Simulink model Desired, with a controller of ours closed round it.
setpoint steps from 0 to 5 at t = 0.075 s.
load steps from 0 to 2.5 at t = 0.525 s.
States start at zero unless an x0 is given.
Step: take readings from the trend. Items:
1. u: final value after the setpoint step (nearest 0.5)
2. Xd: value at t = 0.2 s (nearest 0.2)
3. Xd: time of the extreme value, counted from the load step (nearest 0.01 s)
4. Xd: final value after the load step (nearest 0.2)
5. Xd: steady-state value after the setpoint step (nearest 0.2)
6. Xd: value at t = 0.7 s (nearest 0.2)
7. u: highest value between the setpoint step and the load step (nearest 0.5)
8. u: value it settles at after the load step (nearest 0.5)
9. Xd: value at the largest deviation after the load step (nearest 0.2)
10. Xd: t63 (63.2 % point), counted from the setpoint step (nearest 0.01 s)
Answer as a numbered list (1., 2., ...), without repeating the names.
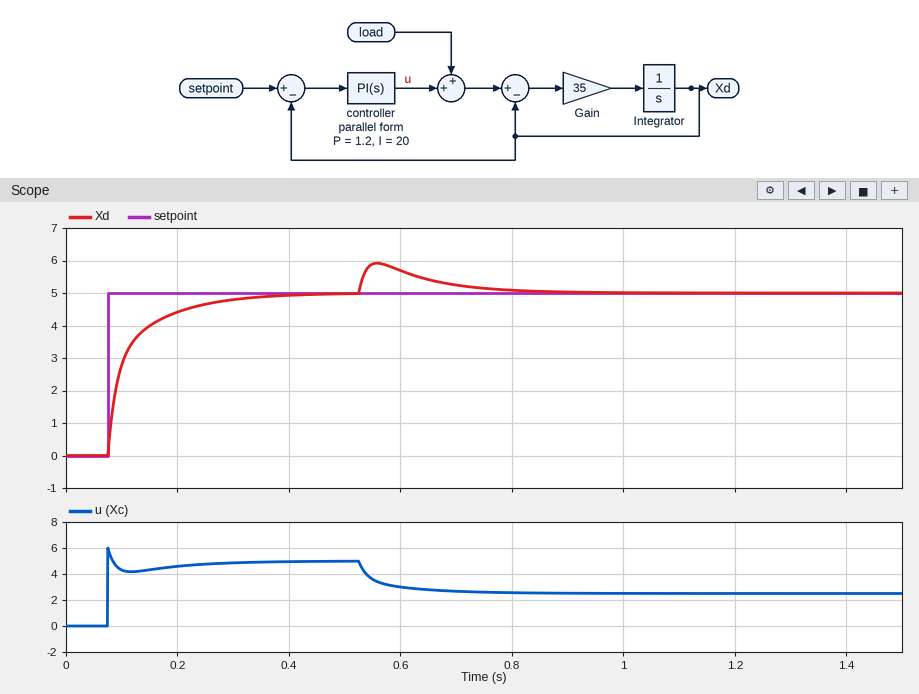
1. 5.0
2. 4.4
3. 0.03 s
4. 5.0
5. 5.0
6. 5.2
7. 6.0
8. 2.5
9. 6.0
10. 0.03 s
